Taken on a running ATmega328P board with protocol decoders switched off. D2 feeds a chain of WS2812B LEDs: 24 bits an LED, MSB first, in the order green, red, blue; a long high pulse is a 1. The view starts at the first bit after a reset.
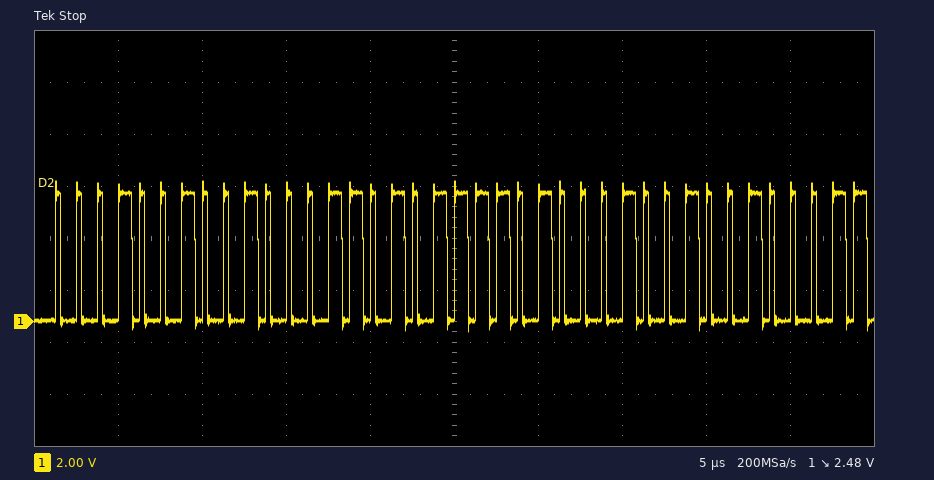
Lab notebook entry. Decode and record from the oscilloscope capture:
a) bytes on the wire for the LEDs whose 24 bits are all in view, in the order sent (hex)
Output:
12 46 BD
